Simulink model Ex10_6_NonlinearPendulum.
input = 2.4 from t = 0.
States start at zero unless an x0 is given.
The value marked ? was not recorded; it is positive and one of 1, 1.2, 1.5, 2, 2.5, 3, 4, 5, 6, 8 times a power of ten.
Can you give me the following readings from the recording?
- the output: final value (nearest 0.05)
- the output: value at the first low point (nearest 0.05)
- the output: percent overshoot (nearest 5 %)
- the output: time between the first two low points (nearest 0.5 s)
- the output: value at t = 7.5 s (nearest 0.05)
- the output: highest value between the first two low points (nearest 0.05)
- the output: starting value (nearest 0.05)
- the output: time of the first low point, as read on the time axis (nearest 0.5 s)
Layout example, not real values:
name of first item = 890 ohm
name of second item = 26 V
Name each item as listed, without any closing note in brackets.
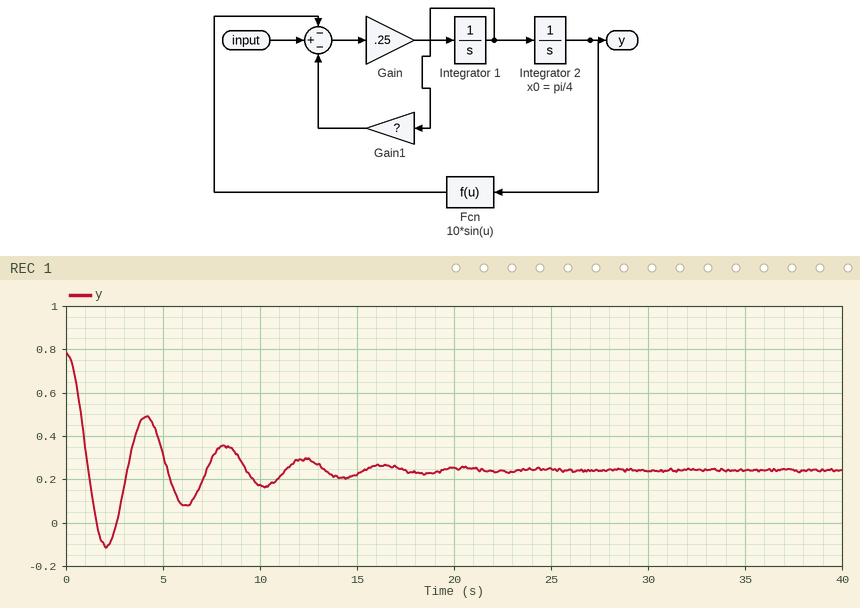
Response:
the output: final value = 0.25
the output: value at the first low point = -0.10
the output: percent overshoot = 65 %
the output: time between the first two low points = 4.0 s
the output: value at t = 7.5 s = 0.30
the output: highest value between the first two low points = 0.50
the output: starting value = 0.80
the output: time of the first low point, as read on the time axis = 2.0 s
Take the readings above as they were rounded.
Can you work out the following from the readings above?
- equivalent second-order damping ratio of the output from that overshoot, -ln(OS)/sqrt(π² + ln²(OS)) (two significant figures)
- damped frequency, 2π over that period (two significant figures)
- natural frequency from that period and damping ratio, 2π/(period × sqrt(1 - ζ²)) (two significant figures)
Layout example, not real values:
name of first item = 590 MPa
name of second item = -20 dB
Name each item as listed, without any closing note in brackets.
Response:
equivalent second-order damping ratio of the output from that overshoot, -ln(OS)/sqrt(π² + ln²(OS)) = 0.14
damped frequency, 2π over that period = 1.6 rad/s
natural frequency from that period and damping ratio, 2π/(period × sqrt(1 - ζ²)) = 1.6 rad/s
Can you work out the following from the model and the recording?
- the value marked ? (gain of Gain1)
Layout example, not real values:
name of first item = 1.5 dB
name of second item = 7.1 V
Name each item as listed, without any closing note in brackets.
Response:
the value marked ? = 1.5
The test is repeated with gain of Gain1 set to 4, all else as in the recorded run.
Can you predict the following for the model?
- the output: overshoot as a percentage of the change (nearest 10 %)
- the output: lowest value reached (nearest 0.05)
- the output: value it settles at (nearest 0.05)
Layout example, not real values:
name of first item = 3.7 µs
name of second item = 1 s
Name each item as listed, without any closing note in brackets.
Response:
the output: overshoot as a percentage of the change = 30 %
the output: lowest value reached = 0.05
the output: value it settles at = 0.25
